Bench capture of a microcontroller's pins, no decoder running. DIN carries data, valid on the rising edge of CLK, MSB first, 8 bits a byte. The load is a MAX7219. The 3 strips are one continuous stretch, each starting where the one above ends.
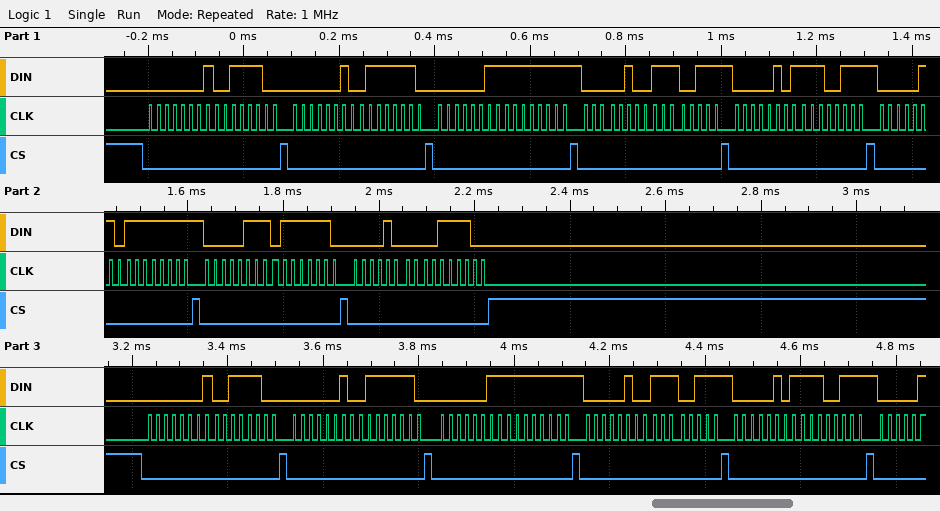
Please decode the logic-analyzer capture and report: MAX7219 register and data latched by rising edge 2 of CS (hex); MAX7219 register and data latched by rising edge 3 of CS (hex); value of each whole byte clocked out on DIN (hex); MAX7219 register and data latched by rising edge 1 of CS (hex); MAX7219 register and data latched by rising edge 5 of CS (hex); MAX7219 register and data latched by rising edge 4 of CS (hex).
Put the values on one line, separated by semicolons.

register 0x2, data 0x7E; register 0x3, data 0xFF; 01 3C 02 7E 03 FF 04 E7 05 E7 06 FF 07 7E 08 3C 01 3C 02 7E 03 FF 04 E7 05 E7; register 0x1, data 0x3C; register 0x5, data 0xE7; register 0x4, data 0xE7
